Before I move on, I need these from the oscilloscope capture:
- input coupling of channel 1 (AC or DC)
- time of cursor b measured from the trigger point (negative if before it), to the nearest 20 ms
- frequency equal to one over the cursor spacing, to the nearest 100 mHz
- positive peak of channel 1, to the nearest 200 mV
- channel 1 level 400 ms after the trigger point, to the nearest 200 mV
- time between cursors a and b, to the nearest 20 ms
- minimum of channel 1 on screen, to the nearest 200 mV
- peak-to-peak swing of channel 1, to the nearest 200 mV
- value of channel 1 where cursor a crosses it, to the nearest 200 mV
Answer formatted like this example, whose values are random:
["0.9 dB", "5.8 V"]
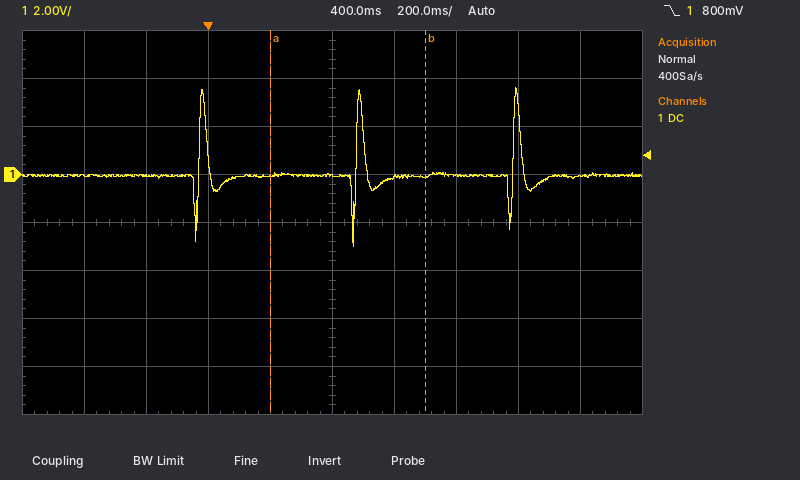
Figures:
["DC", "+700 ms", "2.0 Hz", "3.6 V", "0.0 V", "500 ms", "-3.0 V", "6.6 V", "0.0 V"]
